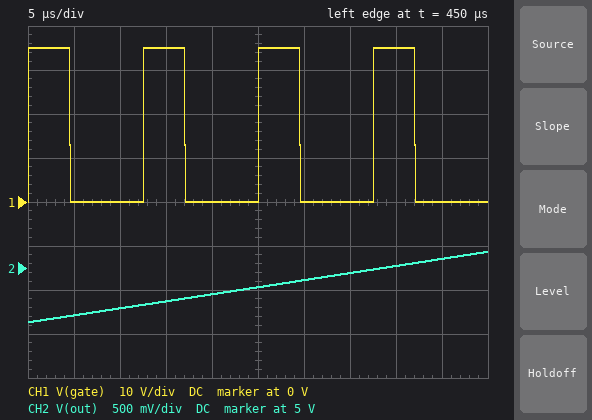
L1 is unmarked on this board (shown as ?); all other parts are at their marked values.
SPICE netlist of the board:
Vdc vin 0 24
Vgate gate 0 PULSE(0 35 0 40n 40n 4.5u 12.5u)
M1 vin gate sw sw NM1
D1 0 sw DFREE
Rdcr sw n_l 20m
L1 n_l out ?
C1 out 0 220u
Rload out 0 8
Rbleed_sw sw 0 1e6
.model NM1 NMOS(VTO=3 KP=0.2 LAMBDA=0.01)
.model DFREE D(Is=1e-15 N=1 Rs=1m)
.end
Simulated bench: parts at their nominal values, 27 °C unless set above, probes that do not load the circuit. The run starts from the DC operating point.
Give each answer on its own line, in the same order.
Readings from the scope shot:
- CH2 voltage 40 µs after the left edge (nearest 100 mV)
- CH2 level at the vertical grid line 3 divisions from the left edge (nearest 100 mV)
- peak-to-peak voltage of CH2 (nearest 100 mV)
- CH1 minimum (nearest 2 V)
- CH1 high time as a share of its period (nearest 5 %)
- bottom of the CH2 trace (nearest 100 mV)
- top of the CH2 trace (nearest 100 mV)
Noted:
5.0 V
4.6 V
800 mV
0 V
35 %
4.4 V
5.2 V
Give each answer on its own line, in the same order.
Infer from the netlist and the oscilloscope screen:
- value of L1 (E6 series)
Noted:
680 µH
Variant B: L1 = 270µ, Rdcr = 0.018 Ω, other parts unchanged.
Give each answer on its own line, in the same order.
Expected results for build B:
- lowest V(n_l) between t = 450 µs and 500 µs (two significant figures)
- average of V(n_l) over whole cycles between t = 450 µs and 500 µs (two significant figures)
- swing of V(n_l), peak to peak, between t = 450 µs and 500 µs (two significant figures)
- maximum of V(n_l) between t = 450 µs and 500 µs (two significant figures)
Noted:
-1.1 V
6.9 V
22 V
21 V
